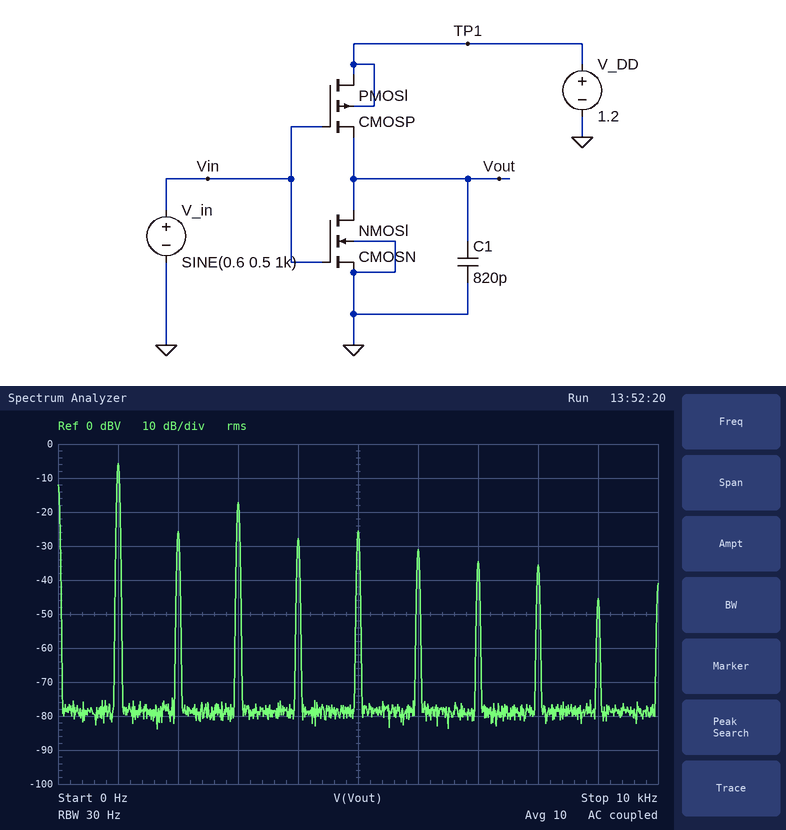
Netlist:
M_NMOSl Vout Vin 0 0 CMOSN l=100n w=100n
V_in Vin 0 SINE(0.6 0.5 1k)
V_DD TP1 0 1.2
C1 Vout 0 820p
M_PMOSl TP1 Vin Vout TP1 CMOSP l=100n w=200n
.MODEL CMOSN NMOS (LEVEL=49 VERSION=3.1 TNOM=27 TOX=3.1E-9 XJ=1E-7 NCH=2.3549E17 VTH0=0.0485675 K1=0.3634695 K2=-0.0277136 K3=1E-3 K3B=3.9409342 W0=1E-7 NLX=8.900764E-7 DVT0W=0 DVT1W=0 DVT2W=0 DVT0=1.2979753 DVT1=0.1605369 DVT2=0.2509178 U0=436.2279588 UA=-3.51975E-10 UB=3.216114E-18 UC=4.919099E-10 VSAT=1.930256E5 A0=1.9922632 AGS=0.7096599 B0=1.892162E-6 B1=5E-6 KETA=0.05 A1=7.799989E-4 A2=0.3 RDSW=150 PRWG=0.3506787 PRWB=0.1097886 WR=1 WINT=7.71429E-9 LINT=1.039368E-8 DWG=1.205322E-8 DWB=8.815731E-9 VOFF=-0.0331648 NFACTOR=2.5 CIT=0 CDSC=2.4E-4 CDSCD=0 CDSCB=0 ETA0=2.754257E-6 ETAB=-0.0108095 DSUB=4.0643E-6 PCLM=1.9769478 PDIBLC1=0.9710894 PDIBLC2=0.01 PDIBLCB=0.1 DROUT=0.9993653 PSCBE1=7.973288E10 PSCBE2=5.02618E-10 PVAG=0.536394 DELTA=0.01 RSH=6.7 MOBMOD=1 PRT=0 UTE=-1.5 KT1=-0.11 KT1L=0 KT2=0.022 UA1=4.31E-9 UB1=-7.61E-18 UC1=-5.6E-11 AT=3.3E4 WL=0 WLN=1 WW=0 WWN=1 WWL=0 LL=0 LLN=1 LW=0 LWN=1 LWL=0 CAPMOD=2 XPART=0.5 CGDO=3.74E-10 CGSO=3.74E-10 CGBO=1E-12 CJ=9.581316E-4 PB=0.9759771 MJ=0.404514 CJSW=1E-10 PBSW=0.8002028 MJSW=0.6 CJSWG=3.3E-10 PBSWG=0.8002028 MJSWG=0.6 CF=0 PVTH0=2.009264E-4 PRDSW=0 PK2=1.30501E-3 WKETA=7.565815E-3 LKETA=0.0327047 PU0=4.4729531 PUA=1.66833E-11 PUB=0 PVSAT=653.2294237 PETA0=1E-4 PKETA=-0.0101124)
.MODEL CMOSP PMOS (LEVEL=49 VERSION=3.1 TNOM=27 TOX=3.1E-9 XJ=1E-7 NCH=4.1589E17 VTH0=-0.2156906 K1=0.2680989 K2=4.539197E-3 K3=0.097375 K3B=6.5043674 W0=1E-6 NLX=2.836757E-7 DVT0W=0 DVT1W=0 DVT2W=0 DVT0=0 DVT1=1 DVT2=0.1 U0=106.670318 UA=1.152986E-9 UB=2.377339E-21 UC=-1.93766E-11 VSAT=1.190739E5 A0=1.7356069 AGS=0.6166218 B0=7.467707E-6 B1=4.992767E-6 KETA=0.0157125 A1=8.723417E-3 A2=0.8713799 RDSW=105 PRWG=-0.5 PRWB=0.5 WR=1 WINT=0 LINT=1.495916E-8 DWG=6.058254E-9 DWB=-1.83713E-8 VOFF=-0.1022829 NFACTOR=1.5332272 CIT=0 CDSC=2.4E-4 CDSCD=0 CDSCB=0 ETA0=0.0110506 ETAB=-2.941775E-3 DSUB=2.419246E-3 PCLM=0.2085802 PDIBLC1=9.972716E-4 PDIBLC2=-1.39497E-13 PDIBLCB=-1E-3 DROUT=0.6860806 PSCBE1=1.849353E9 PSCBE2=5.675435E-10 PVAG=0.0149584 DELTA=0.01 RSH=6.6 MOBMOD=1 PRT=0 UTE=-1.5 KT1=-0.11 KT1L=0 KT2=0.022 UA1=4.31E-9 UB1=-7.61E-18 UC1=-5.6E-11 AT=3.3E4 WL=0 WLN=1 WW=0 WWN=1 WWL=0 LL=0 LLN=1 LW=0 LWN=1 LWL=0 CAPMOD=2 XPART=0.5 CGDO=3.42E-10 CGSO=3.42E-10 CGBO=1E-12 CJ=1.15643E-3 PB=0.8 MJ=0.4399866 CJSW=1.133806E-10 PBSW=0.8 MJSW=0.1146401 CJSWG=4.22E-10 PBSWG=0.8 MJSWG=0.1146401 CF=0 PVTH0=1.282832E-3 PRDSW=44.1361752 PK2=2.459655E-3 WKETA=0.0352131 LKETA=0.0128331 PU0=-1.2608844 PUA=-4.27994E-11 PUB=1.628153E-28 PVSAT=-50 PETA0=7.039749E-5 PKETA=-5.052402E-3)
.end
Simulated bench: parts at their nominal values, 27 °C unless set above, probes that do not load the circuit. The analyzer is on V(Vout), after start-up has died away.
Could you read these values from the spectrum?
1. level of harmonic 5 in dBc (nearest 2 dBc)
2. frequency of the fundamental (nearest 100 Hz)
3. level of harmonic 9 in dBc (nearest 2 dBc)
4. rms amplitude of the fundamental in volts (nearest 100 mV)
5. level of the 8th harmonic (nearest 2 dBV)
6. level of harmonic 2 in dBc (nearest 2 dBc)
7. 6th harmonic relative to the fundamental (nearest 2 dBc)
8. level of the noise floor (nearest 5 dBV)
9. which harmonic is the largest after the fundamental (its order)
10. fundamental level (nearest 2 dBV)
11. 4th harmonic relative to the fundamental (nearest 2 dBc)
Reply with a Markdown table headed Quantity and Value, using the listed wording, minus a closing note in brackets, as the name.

| Quantity | Value |
|---|---|
| level of harmonic 5 in dBc | -20 dBc |
| frequency of the fundamental | 1.0 kHz |
| level of harmonic 9 in dBc | -40 dBc |
| rms amplitude of the fundamental in volts | 500 mV |
| level of the 8th harmonic | -36 dBV |
| level of harmonic 2 in dBc | -20 dBc |
| 6th harmonic relative to the fundamental | -26 dBc |
| level of the noise floor | -80 dBV |
| which harmonic is the largest after the fundamental | 3 |
| fundamental level | -6 dBV |
| 4th harmonic relative to the fundamental | -22 dBc |
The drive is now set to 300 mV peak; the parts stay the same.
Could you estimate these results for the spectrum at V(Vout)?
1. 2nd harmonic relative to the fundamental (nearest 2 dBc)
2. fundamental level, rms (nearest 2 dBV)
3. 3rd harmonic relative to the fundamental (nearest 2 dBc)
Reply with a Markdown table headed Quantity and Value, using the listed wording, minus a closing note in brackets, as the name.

| Quantity | Value |
|---|---|
| 2nd harmonic relative to the fundamental | -18 dBc |
| fundamental level, rms | -6 dBV |
| 3rd harmonic relative to the fundamental | -14 dBc |
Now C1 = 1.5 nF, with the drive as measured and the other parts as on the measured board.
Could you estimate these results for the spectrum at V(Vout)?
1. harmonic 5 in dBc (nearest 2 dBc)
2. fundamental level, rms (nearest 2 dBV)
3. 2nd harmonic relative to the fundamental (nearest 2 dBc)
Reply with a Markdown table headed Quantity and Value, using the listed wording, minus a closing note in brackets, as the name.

| Quantity | Value |
|---|---|
| harmonic 5 in dBc | -24 dBc |
| fundamental level, rms | -6 dBV |
| 2nd harmonic relative to the fundamental | -18 dBc |
